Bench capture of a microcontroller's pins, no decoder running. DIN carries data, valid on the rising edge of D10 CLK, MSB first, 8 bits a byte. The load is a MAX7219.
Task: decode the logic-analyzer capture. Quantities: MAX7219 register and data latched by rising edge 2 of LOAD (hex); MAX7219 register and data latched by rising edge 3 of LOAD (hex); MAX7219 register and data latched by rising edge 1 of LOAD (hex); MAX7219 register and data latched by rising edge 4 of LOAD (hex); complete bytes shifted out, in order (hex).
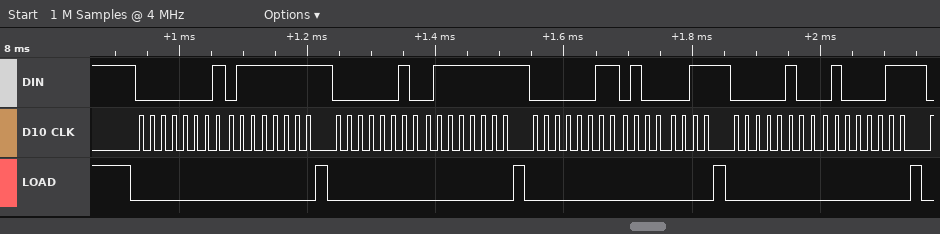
register 0x2, data 0x7F
register 0x3, data 0x43
register 0x1, data 0x7F
register 0x4, data 0x43
0x01 0x7F 0x02 0x7F 0x03 0x43 0x04 0x43
